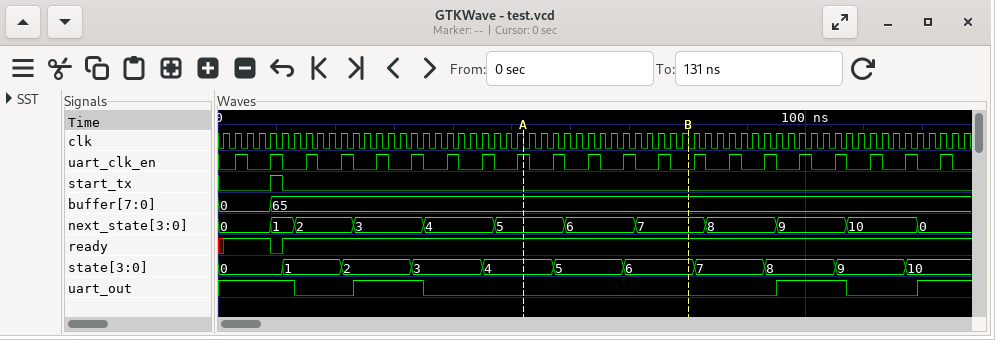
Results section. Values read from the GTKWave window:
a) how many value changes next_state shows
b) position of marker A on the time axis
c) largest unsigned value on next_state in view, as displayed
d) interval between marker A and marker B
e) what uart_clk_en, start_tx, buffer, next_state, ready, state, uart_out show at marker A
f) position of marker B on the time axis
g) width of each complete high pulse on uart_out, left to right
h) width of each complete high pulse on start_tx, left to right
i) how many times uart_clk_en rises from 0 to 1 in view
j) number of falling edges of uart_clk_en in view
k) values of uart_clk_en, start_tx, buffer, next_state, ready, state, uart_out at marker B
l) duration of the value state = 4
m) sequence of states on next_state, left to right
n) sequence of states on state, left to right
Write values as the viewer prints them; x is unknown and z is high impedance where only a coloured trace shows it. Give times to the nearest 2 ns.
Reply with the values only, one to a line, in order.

11
52 ns
10
28 ns
uart_clk_en=1, start_tx=0, buffer=65, next_state=5, ready=1, state=4, uart_out=0
80 ns
12 ns, 12 ns
2 ns
21
21
uart_clk_en=0, start_tx=0, buffer=65, next_state=7, ready=1, state=6, uart_out=0
12 ns
0, 1, 2, 3, 4, 5, 6, 7, 8, 9, 10, 0
0, 1, 2, 3, 4, 5, 6, 7, 8, 9, 10
